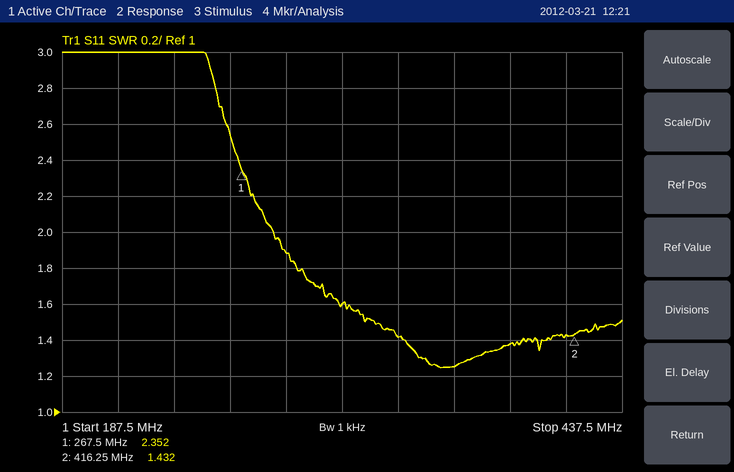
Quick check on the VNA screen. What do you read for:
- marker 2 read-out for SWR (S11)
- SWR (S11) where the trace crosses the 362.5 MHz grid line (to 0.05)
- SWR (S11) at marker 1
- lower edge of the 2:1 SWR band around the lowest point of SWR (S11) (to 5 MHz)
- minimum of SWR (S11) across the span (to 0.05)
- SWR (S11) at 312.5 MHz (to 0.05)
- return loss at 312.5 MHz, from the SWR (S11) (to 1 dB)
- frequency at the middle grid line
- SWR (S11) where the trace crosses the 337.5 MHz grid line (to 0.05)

1.432
1.25
2.352
280 MHz
1.25
1.60
13 dB
312.5 MHz
1.40
